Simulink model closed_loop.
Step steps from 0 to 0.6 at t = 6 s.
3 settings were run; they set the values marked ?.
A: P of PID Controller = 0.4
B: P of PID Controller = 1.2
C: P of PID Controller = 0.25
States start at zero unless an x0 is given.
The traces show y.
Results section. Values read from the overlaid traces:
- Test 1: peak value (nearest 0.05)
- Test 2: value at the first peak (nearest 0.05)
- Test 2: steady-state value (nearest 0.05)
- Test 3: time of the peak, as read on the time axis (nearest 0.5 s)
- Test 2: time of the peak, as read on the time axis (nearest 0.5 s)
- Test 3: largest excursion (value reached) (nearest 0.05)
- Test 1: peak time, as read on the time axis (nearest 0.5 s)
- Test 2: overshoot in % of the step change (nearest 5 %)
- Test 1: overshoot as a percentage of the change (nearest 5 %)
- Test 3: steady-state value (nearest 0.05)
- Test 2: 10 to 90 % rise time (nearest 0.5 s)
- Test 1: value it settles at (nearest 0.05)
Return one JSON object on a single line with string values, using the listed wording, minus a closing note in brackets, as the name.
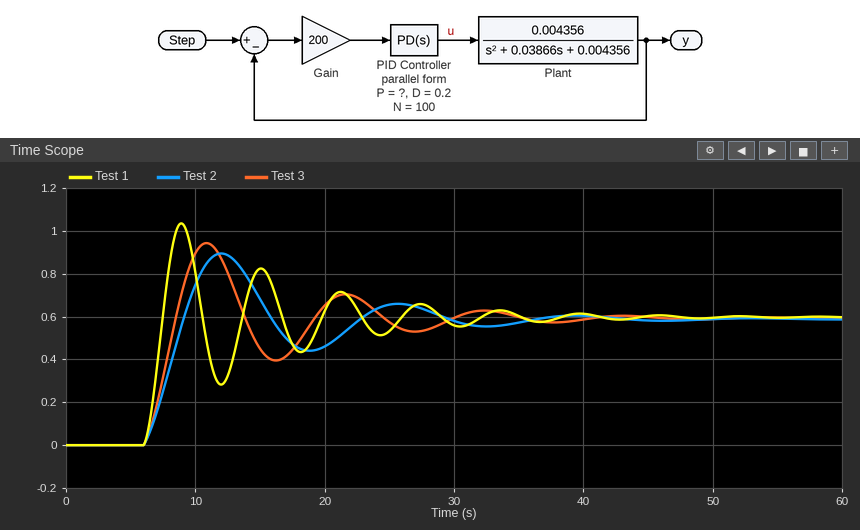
{"Test 1: peak value": "1.05", "Test 2: value at the first peak": "0.90", "Test 2: steady-state value": "0.60", "Test 3: time of the peak, as read on the time axis": "11.0 s", "Test 2: time of the peak, as read on the time axis": "12.0 s", "Test 3: largest excursion (value reached)": "0.95", "Test 1: peak time, as read on the time axis": "9.0 s", "Test 2: overshoot in % of the step change": "50 %", "Test 1: overshoot as a percentage of the change": "75 %", "Test 3: steady-state value": "0.60", "Test 2: 10 to 90 % rise time": "2.5 s", "Test 1: value it settles at": "0.60"}
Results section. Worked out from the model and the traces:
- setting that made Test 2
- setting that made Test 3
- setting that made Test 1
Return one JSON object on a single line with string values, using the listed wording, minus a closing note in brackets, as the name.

{"setting that made Test 2": "C", "setting that made Test 3": "A", "setting that made Test 1": "B"}
